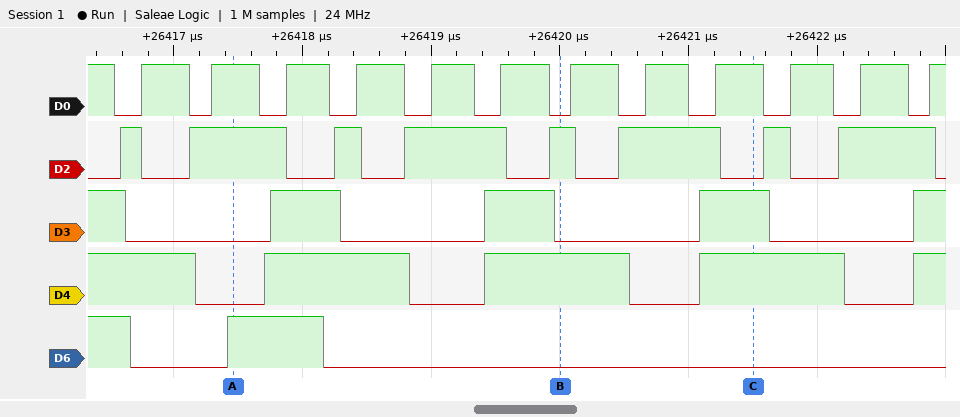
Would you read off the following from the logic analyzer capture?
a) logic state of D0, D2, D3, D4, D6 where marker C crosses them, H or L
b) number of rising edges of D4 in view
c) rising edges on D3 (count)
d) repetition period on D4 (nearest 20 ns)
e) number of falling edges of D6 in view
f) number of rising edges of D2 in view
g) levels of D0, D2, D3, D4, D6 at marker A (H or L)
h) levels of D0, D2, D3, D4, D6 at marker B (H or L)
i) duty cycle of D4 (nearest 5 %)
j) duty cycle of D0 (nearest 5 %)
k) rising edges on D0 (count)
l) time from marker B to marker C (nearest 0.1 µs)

D0=H, D2=L, D3=H, D4=H, D6=L
4
4
1680 ns
2
8
D0=H, D2=H, D3=L, D4=L, D6=H
D0=L, D2=H, D3=L, D4=H, D6=L
65 %
65 %
12
1.5 µs
